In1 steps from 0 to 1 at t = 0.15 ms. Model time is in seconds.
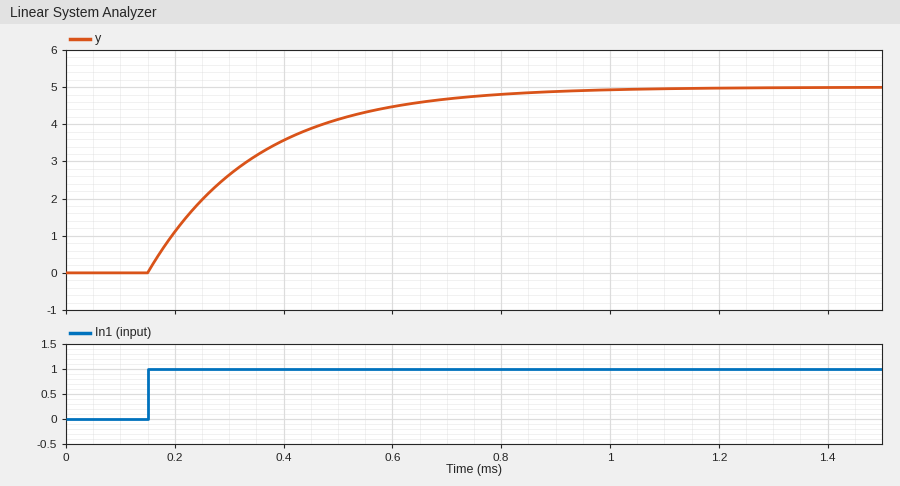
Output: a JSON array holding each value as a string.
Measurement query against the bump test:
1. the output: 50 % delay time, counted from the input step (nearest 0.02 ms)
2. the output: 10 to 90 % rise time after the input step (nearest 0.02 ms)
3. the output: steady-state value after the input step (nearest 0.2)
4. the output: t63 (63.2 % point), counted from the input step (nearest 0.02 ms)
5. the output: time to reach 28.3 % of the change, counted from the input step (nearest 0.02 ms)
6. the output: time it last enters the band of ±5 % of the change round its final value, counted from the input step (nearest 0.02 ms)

["0.14 ms", "0.44 ms", "5.0", "0.20 ms", "0.06 ms", "0.60 ms"]
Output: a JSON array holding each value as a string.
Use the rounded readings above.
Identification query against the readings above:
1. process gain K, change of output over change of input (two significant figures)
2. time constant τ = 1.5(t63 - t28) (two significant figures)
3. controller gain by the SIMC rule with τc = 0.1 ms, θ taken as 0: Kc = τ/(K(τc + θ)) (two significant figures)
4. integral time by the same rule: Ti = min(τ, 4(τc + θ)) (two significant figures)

["5.0", "0.21 ms", "0.42", "0.21 ms"]
